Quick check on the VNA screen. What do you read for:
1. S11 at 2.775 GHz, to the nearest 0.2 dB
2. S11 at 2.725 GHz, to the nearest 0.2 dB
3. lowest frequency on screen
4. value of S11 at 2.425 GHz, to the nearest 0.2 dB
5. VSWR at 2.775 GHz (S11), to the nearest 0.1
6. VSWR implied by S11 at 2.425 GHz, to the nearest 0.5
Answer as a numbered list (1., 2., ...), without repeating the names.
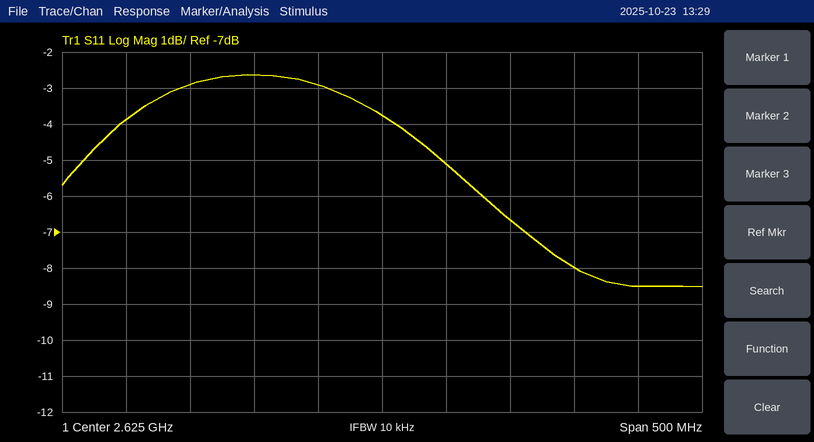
1. -8.0 dB
2. -6.6 dB
3. 2.375 GHz
4. -3.8 dB
5. 2.3
6. 4.5
